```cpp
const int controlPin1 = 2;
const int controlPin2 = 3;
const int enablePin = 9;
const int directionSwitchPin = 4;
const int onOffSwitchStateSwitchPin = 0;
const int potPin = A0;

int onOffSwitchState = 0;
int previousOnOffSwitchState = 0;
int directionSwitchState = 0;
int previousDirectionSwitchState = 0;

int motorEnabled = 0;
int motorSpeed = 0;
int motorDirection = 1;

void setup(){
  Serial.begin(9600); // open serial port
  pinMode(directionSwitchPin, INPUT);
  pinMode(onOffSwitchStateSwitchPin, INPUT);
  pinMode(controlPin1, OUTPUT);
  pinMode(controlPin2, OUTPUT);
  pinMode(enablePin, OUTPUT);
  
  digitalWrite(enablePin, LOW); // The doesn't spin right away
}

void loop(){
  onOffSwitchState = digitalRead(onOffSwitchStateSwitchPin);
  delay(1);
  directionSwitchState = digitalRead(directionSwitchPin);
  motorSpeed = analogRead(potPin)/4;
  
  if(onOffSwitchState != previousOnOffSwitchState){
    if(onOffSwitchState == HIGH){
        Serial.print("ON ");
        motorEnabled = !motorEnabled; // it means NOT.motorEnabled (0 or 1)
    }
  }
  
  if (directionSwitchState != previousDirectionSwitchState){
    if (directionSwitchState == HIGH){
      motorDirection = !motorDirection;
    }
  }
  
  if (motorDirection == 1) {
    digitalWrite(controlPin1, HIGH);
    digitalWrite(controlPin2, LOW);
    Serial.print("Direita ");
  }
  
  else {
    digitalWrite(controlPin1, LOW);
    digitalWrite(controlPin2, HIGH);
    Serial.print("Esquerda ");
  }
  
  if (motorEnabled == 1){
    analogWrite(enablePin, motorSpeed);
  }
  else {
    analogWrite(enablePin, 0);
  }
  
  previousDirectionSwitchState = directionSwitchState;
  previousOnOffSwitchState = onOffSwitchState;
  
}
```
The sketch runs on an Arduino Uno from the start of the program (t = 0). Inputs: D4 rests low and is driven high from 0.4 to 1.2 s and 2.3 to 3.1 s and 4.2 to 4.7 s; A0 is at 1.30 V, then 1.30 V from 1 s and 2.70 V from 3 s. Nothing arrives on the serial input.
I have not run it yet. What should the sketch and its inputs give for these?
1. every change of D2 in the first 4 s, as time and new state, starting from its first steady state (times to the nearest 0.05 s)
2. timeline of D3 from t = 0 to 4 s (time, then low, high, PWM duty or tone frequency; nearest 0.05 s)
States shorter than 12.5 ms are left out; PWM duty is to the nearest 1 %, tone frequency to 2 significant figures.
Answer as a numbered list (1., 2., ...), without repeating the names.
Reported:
1. 0 s high; 0.4 s low; 2.3 s high
2. 0 s low; 0.4 s high; 2.3 s low
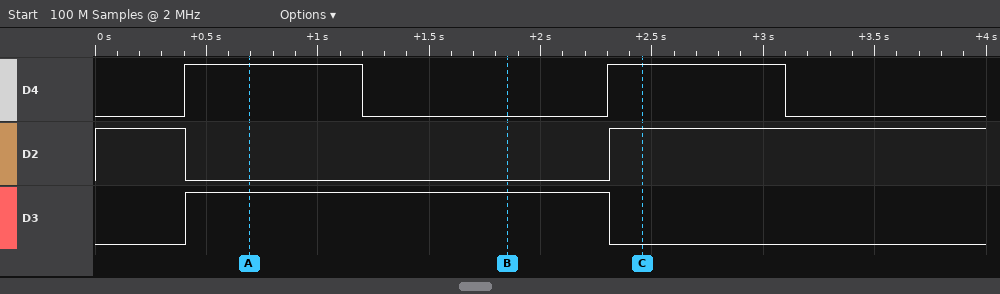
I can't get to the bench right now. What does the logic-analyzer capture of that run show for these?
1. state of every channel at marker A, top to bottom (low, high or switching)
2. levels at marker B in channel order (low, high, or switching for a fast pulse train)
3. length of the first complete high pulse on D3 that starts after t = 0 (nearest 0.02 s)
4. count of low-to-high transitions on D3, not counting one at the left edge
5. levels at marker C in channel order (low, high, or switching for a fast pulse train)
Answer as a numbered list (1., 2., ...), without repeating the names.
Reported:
1. D4 high, D2 low, D3 high
2. D4 low, D2 low, D3 high
3. 1.90 s
4. 1
5. D4 high, D2 high, D3 low
